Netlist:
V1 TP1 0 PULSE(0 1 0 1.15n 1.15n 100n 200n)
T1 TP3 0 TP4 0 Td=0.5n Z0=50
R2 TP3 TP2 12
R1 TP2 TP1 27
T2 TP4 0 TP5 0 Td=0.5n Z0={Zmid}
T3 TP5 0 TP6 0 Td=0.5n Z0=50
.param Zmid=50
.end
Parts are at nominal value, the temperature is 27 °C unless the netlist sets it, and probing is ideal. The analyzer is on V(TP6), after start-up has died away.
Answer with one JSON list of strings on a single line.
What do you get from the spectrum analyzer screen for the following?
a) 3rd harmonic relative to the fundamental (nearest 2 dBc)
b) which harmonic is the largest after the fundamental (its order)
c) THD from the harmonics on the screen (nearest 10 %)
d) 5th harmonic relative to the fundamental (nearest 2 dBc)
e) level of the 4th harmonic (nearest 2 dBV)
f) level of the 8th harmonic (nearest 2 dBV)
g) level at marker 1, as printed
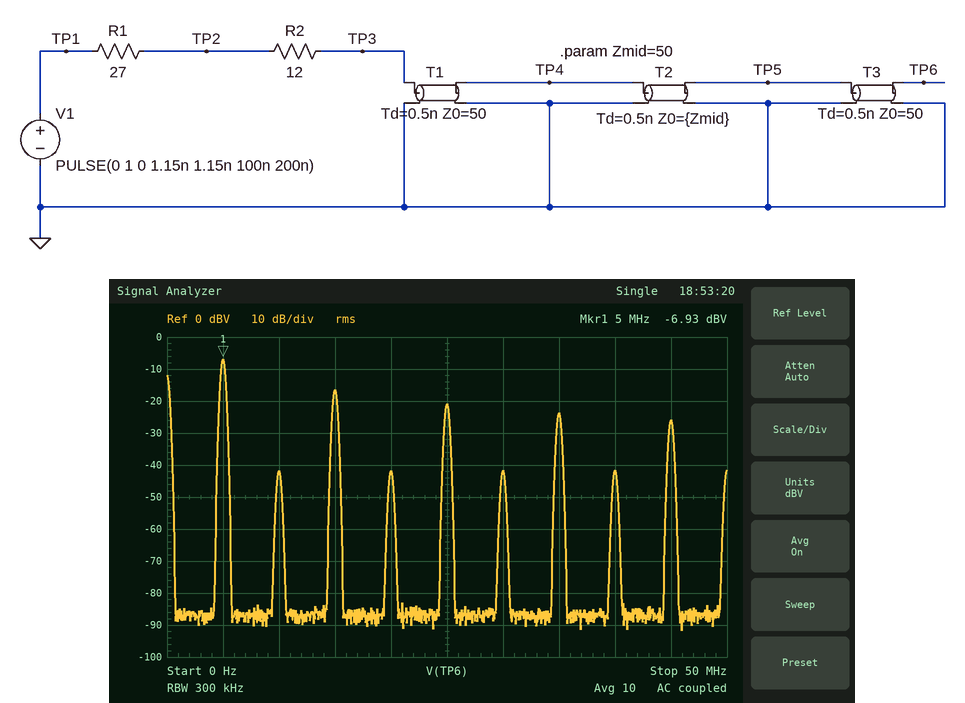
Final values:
["-10 dBc", "3", "40 %", "-14 dBc", "-42 dBV", "-42 dBV", "-6.93 dBV"]
